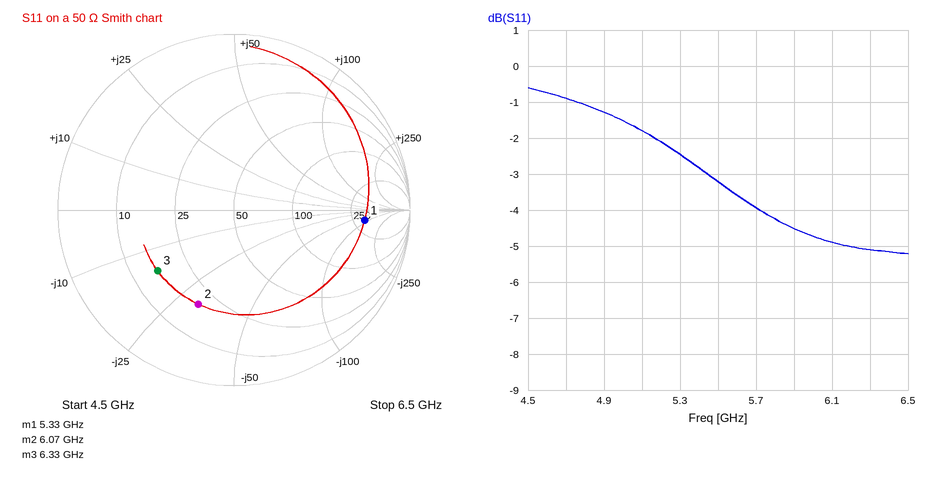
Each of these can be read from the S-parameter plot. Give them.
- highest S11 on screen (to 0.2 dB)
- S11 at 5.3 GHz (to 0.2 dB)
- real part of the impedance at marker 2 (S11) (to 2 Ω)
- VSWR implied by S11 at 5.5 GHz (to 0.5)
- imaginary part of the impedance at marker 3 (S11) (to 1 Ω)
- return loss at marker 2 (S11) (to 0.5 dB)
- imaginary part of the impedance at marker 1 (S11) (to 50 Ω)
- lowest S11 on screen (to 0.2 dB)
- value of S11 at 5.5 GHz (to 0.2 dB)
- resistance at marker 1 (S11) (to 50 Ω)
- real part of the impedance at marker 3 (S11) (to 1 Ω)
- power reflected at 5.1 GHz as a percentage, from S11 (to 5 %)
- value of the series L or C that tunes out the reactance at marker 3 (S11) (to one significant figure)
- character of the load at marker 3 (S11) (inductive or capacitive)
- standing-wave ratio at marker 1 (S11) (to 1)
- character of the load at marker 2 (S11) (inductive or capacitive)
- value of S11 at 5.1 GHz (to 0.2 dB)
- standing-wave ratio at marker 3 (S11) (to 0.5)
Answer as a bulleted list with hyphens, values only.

- -0.6 dB
- -2.4 dB
- 20 Ω
- 5.5
- -16 Ω
- 5.0 dB
- -100 Ω
- -5.2 dB
- -3.2 dB
- 300 Ω
- 16 Ω
- 65 %
- 400 pH
- capacitive
- 7
- capacitive
- -1.8 dB
- 3.5
